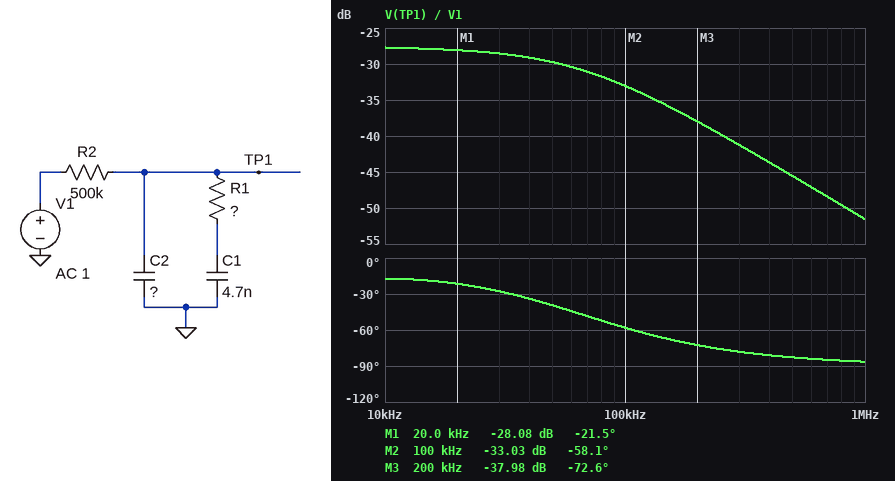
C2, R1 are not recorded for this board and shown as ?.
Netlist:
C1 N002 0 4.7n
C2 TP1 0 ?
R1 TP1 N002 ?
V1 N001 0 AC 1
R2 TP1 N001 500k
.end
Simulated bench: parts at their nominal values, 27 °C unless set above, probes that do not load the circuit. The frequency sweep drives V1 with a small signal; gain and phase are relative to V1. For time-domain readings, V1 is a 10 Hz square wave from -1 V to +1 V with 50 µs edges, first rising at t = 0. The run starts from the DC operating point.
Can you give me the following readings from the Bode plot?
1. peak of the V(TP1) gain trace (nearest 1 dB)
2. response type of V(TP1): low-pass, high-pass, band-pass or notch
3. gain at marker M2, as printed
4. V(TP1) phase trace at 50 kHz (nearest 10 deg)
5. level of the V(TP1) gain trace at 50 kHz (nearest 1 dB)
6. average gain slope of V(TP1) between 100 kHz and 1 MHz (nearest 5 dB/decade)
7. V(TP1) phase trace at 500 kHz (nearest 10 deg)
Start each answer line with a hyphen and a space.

- -28 dB
- low-pass
- -33.03 dB
- -40 deg
- -30 dB
- -20 dB/decade
- -80 deg
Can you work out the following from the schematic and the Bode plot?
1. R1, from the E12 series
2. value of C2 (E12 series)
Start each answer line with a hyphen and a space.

- 22 kΩ
- 120 pF
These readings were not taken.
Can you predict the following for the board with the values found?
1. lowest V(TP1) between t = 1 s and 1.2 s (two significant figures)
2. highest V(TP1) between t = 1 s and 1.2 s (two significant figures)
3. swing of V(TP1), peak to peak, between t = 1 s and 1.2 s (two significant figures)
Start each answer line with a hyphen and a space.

- -1.0 V
- 1.0 V
- 2.0 V
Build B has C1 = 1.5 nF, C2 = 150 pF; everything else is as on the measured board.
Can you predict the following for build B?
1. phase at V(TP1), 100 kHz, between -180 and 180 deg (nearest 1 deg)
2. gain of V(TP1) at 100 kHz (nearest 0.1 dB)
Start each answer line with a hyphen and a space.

- -64 deg
- -34.6 dB
